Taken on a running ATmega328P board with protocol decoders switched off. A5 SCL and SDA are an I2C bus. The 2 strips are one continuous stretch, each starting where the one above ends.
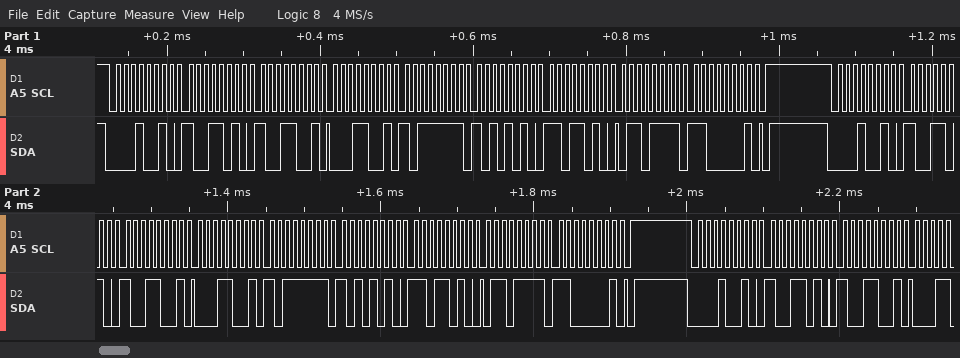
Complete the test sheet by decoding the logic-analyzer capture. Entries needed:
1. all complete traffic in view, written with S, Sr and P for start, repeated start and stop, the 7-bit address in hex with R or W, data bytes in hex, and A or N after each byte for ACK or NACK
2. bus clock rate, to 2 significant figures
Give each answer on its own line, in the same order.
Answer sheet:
S 09W A 9A A 99 A 19 A BF A AA A DA A 6F A C1 A P S 09W A 9A A 99 A 19 A BF A AA A DA A 6F A C1 A P S 09W A 9A A 99 A
100 kHz
